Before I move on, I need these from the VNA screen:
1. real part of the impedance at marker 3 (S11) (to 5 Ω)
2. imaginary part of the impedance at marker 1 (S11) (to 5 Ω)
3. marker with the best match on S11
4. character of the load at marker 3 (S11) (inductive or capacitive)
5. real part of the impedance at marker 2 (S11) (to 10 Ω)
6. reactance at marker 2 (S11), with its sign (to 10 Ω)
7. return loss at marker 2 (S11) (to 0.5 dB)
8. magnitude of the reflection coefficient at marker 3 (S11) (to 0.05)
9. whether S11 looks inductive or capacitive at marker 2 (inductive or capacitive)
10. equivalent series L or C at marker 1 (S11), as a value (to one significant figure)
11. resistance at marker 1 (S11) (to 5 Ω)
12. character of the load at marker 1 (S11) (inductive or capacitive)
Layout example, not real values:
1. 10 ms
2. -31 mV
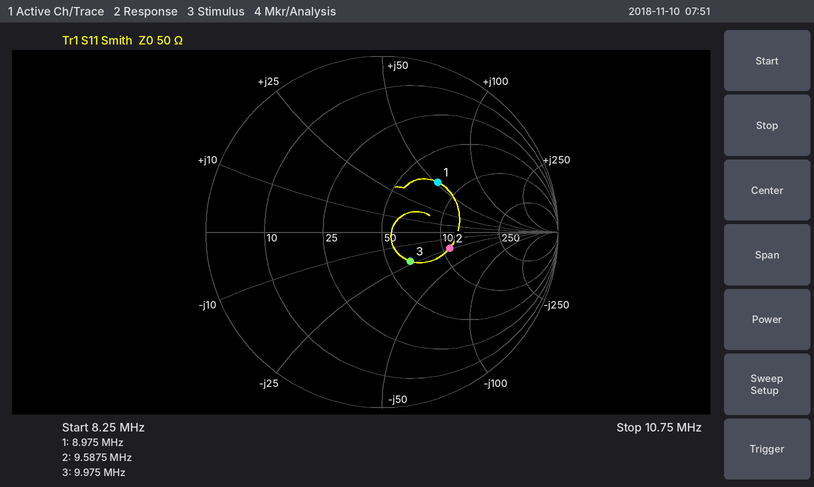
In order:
1. 65 Ω
2. +50 Ω
3. marker 3
4. capacitive
5. 110 Ω
6. -20 Ω
7. 8.0 dB
8. 0.25
9. capacitive
10. 900 nH
11. 75 Ω
12. inductive
